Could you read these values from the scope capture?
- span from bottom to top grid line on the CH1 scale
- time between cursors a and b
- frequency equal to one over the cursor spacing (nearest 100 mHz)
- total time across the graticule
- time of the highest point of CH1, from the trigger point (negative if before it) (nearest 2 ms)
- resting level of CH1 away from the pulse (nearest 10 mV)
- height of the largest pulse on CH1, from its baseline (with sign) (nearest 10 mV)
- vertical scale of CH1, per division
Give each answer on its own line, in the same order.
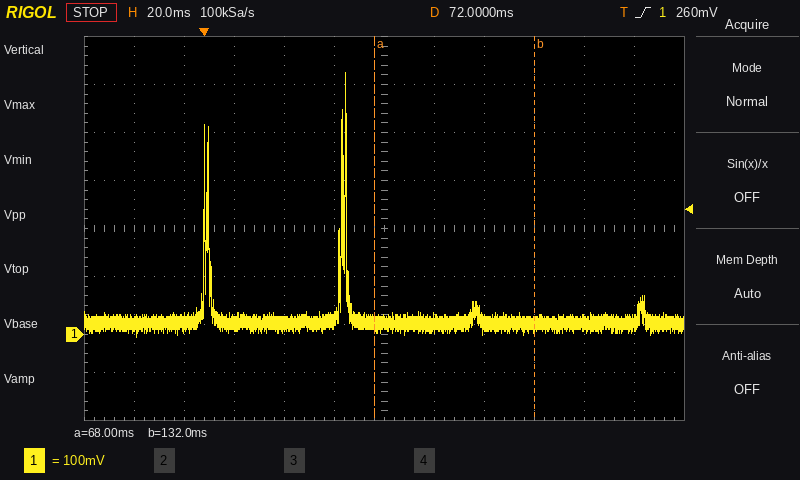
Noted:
800 mV
64 ms
15.6 Hz
240 ms
+56 ms
20 mV
+520 mV
100 mV
